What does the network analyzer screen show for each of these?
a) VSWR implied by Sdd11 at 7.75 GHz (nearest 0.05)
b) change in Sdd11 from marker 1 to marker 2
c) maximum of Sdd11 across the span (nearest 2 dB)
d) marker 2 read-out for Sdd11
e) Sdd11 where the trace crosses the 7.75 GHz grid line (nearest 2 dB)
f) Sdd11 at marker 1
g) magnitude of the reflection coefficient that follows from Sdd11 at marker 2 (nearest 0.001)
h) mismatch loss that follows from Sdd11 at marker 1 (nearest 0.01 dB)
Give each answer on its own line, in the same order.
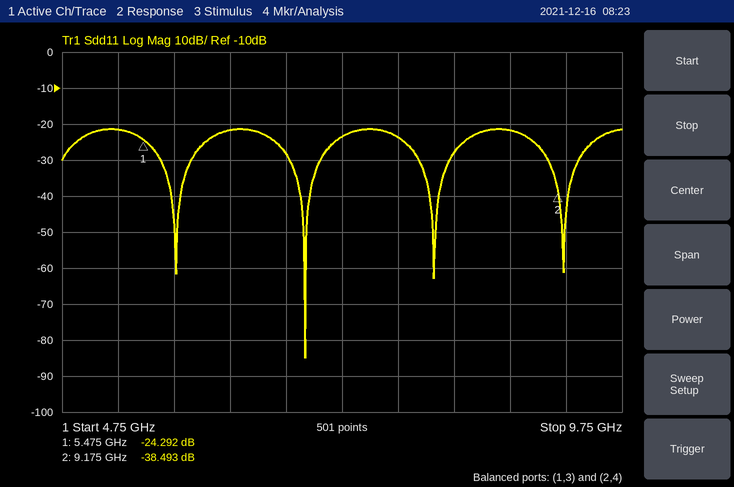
1.15
-14.201 dB
-22 dB
-38.493 dB
-24 dB
-24.292 dB
0.012
0.02 dB
